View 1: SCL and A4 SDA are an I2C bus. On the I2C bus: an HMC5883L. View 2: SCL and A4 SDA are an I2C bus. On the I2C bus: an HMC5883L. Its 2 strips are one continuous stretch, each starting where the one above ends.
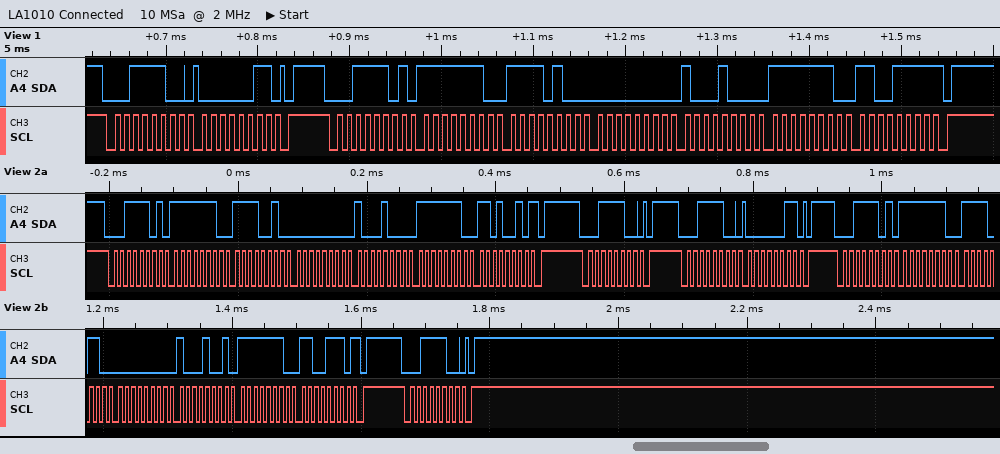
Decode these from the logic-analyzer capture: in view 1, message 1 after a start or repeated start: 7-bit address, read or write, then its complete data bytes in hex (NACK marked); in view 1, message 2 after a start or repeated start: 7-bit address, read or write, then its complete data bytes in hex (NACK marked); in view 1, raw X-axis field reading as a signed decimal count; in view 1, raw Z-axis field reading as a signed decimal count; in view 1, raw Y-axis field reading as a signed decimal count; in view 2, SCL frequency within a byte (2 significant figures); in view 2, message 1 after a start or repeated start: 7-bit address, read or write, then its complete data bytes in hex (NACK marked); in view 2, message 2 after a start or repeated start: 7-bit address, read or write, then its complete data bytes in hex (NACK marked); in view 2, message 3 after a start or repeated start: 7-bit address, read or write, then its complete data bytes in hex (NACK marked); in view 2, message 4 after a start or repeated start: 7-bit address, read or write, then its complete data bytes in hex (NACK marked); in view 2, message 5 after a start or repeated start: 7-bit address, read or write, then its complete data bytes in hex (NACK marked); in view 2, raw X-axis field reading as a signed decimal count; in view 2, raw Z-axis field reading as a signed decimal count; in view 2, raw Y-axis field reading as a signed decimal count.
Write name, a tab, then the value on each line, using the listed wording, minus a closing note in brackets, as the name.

in view 1, message 1 after a start or repeated start: 7-bit address, read or write, then its complete data bytes in hex	0x1E write: 03
in view 1, message 2 after a start or repeated start: 7-bit address, read or write, then its complete data bytes in hex	0x1E read: FE F4 00 88 FE CF NACK
in view 1, raw X-axis field reading as a signed decimal count	-268
in view 1, raw Z-axis field reading as a signed decimal count	136
in view 1, raw Y-axis field reading as a signed decimal count	-305
in view 2, SCL frequency within a byte	100 kHz
in view 2, message 1 after a start or repeated start: 7-bit address, read or write, then its complete data bytes in hex	0x1E read: FE F2 00 88 FE D2 NACK
in view 2, message 2 after a start or repeated start: 7-bit address, read or write, then its complete data bytes in hex	0x1E write
in view 2, message 3 after a start or repeated start: 7-bit address, read or write, then its complete data bytes in hex	0x1E write: 03
in view 2, message 4 after a start or repeated start: 7-bit address, read or write, then its complete data bytes in hex	0x1E read: FE F6 00 89 FE CE NACK
in view 2, message 5 after a start or repeated start: 7-bit address, read or write, then its complete data bytes in hex	0x1E write
in view 2, raw X-axis field reading as a signed decimal count	-266
in view 2, raw Z-axis field reading as a signed decimal count	137
in view 2, raw Y-axis field reading as a signed decimal count	-306
